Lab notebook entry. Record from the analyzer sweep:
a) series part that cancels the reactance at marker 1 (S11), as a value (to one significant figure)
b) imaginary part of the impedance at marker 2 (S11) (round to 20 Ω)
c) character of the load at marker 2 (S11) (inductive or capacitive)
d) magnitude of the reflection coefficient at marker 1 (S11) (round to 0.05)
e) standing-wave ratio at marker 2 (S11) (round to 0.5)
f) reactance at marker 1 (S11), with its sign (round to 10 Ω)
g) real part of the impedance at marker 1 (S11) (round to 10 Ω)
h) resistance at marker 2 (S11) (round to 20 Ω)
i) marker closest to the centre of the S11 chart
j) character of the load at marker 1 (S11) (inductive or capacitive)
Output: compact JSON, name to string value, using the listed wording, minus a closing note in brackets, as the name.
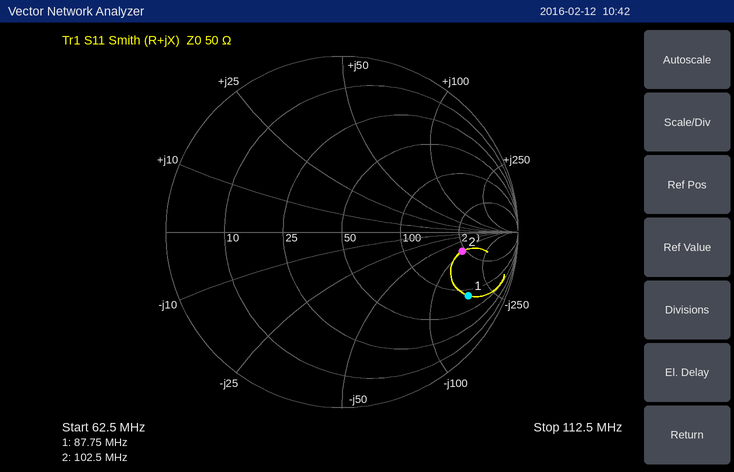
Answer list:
{"series part that cancels the reactance at marker 1 (S11), as a value": "300 nH", "imaginary part of the impedance at marker 2 (S11)": "-100 Ω", "character of the load at marker 2 (S11)": "capacitive", "magnitude of the reflection coefficient at marker 1 (S11)": "0.80", "standing-wave ratio at marker 2 (S11)": "5.5", "reactance at marker 1 (S11), with its sign": "-170 Ω", "real part of the impedance at marker 1 (S11)": "80 Ω", "resistance at marker 2 (S11)": "240 Ω", "marker closest to the centre of the S11 chart": "marker 2", "character of the load at marker 1 (S11)": "capacitive"}
